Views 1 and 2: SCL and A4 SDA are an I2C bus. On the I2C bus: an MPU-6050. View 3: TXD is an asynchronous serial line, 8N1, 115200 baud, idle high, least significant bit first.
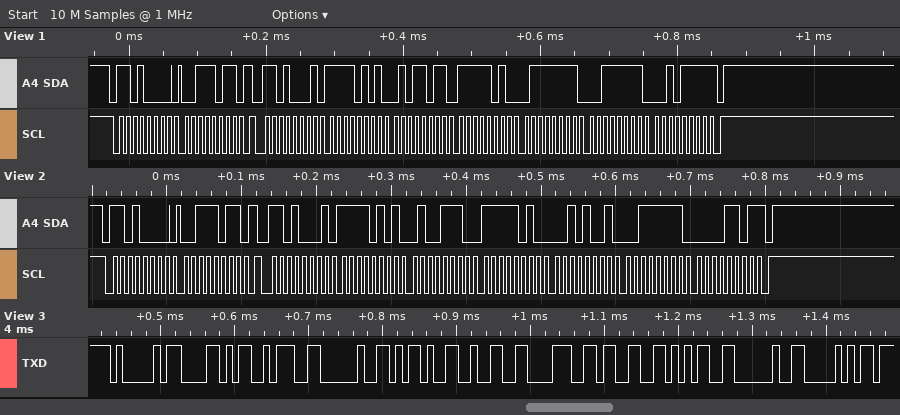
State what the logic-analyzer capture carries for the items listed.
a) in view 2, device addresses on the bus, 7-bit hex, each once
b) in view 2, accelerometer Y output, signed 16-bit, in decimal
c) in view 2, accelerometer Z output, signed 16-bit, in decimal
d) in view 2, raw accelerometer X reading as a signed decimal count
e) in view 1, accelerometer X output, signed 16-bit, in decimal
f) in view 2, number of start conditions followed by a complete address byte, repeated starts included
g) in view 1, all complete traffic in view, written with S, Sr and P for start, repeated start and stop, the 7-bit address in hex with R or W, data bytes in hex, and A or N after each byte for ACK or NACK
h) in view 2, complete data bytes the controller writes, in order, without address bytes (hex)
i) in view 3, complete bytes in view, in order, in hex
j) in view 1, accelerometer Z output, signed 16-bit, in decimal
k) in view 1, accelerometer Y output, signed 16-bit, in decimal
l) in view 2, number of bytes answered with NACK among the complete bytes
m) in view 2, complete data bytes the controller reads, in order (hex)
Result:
0x68
-1495
16141
-2738
-2725
2
S 68W A 3B A Sr 68R A F5 A 5B A FA A 7F A 3F A 2F N P
3B
41 58 3A 20 2D 32 38 33 35 20 50
16175
-1409
1
F5 4E FA 29 3F 0D
